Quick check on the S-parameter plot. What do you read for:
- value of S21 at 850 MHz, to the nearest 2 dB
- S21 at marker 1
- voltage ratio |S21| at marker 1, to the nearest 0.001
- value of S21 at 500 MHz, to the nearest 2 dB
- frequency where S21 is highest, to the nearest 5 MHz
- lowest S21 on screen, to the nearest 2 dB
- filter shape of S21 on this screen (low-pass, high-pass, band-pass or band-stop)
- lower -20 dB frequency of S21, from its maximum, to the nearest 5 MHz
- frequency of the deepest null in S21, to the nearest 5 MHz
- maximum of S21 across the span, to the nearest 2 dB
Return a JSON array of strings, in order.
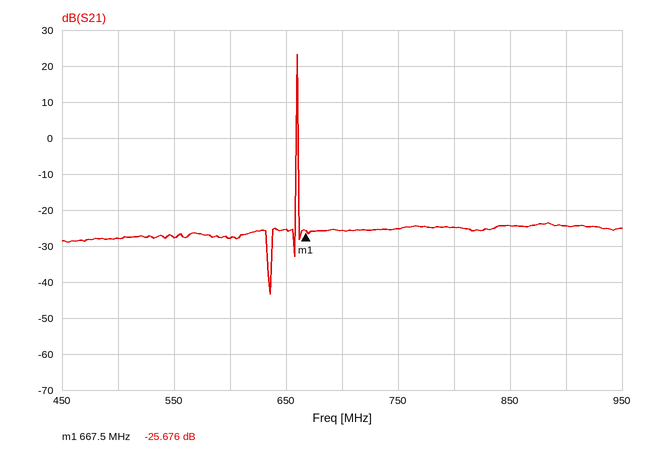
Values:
["-24 dB", "-25.676 dB", "0.052", "-28 dB", "660 MHz", "-44 dB", "band-pass", "660 MHz", "635 MHz", "24 dB"]
